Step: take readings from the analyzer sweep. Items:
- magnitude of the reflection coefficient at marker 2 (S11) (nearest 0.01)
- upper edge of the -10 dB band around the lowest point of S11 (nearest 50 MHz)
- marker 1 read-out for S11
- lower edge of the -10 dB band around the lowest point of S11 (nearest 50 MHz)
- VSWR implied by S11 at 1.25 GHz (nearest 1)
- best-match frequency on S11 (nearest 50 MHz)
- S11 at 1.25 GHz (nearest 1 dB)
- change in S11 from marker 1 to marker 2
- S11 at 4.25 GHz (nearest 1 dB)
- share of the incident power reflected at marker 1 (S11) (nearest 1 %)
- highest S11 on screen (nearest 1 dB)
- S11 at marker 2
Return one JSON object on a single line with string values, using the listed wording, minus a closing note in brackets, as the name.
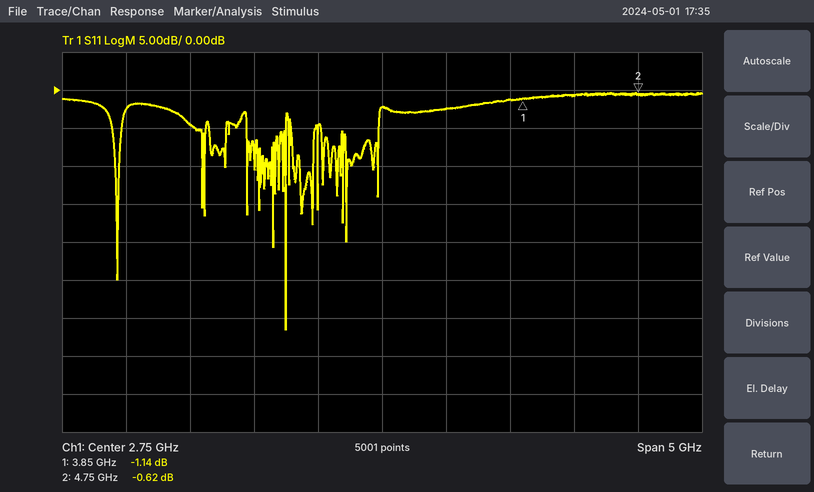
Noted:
{"magnitude of the reflection coefficient at marker 2 (S11)": "0.93", "upper edge of the -10 dB band around the lowest point of S11": "2.00 GHz", "marker 1 read-out for S11": "-1.14 dB", "lower edge of the -10 dB band around the lowest point of S11": "2.00 GHz", "VSWR implied by S11 at 1.25 GHz": "4", "best-match frequency on S11": "2.00 GHz", "S11 at 1.25 GHz": "-5 dB", "change in S11 from marker 1 to marker 2": "0.52 dB", "S11 at 4.25 GHz": "-1 dB", "share of the incident power reflected at marker 1 (S11)": "77 %", "highest S11 on screen": "0 dB", "S11 at marker 2": "-0.62 dB"}
